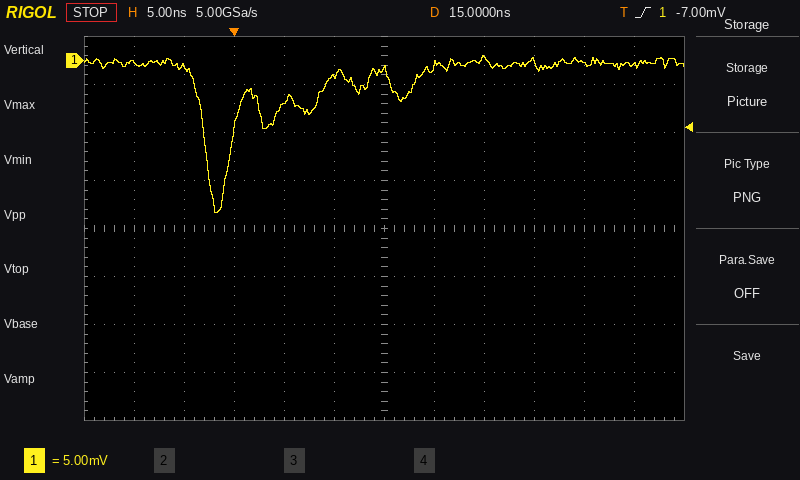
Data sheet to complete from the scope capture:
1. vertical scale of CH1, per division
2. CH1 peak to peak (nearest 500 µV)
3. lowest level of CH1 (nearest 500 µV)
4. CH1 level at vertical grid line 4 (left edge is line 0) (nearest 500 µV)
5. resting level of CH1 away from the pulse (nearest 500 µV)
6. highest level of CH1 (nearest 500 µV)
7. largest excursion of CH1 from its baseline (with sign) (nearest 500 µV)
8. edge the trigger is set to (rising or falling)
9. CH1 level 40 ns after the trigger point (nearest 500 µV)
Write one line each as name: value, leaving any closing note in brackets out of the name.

vertical scale of CH1, per division: 5 mV
CH1 peak to peak: 16.5 mV
lowest level of CH1: -16.0 mV
CH1 level at vertical grid line 4 (left edge is line 0): -4.5 mV
resting level of CH1 away from the pulse: -500 µV
highest level of CH1: 500 µV
largest excursion of CH1 from its baseline (with sign): -15.5 mV
edge the trigger is set to: rising
CH1 level 40 ns after the trigger point: -500 µV
